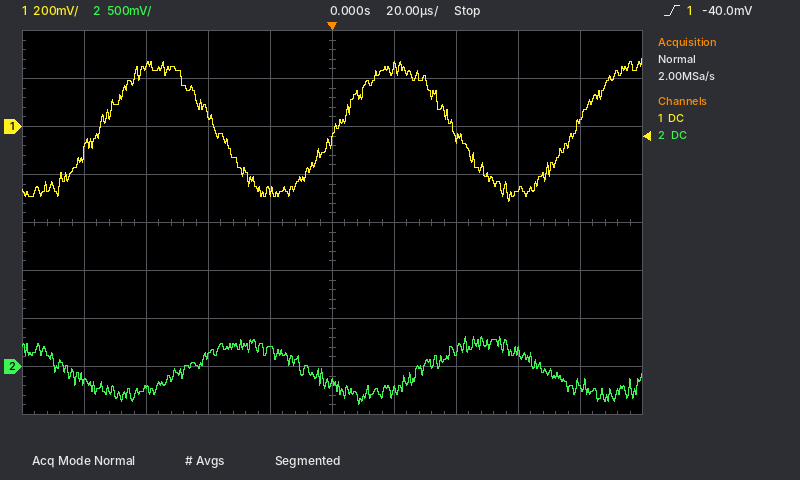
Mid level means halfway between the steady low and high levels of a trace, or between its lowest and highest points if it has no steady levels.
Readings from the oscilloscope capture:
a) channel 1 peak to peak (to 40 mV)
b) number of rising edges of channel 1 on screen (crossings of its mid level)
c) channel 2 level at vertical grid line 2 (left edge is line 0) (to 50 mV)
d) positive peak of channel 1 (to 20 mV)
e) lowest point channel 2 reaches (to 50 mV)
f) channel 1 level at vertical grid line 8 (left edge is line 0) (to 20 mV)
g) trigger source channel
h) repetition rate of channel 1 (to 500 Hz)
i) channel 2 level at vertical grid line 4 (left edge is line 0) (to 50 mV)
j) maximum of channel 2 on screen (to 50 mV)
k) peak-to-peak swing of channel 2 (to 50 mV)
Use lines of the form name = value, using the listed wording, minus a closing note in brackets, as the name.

channel 1 peak to peak = 600 mV
number of rising edges of channel 1 on screen = 3
channel 2 level at vertical grid line 2 (left edge is line 0) = -250 mV
positive peak of channel 1 = 280 mV
lowest point channel 2 reaches = -400 mV
channel 1 level at vertical grid line 8 (left edge is line 0) = -260 mV
trigger source channel = channel 1
repetition rate of channel 1 = 13.0 kHz
channel 2 level at vertical grid line 4 (left edge is line 0) = 200 mV
maximum of channel 2 on screen = 300 mV
peak-to-peak swing of channel 2 = 700 mV
